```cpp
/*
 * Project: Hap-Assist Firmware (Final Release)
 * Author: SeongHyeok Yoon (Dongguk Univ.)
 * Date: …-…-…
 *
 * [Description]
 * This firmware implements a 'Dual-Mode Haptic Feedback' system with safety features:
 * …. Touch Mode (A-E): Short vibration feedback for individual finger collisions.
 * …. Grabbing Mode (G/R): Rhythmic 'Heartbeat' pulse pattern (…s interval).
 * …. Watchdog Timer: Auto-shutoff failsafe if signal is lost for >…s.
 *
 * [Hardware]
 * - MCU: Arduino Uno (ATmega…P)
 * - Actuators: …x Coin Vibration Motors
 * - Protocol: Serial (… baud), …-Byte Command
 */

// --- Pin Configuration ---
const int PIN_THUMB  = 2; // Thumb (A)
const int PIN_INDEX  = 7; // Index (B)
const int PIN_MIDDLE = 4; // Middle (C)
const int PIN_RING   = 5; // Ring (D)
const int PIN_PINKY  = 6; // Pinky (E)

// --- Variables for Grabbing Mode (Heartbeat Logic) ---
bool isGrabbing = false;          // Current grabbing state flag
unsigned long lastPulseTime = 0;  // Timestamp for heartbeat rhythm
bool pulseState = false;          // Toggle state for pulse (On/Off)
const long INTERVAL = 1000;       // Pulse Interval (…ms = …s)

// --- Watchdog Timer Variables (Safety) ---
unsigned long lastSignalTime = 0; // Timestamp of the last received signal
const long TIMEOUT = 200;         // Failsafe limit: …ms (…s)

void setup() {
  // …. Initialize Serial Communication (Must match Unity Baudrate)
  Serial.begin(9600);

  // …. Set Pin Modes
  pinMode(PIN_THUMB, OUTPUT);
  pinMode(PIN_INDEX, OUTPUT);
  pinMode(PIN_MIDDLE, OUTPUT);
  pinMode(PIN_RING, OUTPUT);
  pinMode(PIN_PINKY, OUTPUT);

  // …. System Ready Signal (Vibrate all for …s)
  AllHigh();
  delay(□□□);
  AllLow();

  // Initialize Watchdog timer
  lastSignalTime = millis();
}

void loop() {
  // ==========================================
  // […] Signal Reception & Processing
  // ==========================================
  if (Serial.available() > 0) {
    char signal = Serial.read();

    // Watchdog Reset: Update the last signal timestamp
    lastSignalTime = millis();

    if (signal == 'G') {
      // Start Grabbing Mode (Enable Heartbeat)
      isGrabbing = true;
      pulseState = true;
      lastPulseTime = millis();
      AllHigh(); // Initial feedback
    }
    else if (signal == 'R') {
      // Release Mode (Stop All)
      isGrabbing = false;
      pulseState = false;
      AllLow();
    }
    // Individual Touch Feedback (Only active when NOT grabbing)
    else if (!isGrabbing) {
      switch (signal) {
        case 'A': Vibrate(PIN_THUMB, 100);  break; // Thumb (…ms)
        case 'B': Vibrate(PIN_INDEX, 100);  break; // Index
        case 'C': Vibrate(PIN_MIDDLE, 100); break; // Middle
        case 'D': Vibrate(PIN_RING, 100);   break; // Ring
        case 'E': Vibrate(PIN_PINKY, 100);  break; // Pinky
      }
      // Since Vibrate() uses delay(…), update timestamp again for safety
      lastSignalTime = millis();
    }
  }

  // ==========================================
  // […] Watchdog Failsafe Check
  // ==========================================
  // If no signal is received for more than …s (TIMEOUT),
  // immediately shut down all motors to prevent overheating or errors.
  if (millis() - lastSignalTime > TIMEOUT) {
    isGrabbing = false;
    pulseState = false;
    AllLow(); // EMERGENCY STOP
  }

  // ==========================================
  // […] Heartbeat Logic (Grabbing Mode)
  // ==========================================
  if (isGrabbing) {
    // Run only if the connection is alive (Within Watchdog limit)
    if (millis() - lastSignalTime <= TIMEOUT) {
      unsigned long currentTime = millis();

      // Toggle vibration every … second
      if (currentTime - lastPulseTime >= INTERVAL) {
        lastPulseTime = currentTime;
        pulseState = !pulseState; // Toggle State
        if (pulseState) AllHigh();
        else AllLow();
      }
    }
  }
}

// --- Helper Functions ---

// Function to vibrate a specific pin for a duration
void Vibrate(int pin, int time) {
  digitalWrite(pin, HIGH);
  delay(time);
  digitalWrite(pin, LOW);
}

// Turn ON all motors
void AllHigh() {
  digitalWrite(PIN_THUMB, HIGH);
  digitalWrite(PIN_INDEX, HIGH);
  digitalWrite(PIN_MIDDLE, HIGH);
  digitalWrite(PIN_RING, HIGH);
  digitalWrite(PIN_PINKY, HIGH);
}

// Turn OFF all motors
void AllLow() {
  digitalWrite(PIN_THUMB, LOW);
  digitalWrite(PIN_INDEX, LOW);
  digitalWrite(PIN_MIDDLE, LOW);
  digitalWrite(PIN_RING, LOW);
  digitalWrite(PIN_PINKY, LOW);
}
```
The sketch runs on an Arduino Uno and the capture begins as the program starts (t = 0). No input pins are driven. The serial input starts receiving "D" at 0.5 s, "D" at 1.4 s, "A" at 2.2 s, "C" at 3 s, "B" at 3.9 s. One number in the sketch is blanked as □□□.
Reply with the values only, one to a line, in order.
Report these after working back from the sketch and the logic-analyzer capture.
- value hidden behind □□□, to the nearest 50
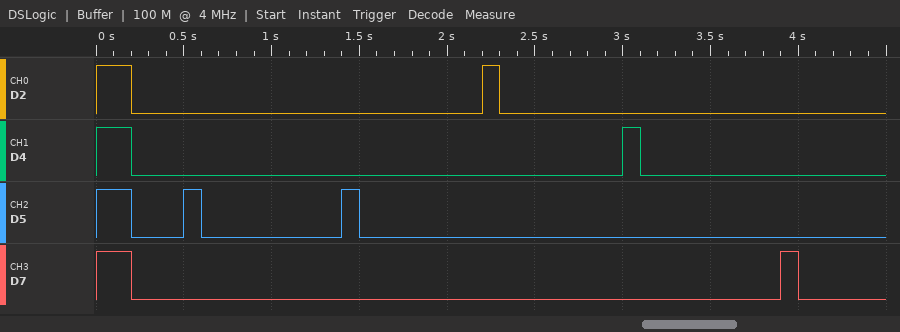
200
